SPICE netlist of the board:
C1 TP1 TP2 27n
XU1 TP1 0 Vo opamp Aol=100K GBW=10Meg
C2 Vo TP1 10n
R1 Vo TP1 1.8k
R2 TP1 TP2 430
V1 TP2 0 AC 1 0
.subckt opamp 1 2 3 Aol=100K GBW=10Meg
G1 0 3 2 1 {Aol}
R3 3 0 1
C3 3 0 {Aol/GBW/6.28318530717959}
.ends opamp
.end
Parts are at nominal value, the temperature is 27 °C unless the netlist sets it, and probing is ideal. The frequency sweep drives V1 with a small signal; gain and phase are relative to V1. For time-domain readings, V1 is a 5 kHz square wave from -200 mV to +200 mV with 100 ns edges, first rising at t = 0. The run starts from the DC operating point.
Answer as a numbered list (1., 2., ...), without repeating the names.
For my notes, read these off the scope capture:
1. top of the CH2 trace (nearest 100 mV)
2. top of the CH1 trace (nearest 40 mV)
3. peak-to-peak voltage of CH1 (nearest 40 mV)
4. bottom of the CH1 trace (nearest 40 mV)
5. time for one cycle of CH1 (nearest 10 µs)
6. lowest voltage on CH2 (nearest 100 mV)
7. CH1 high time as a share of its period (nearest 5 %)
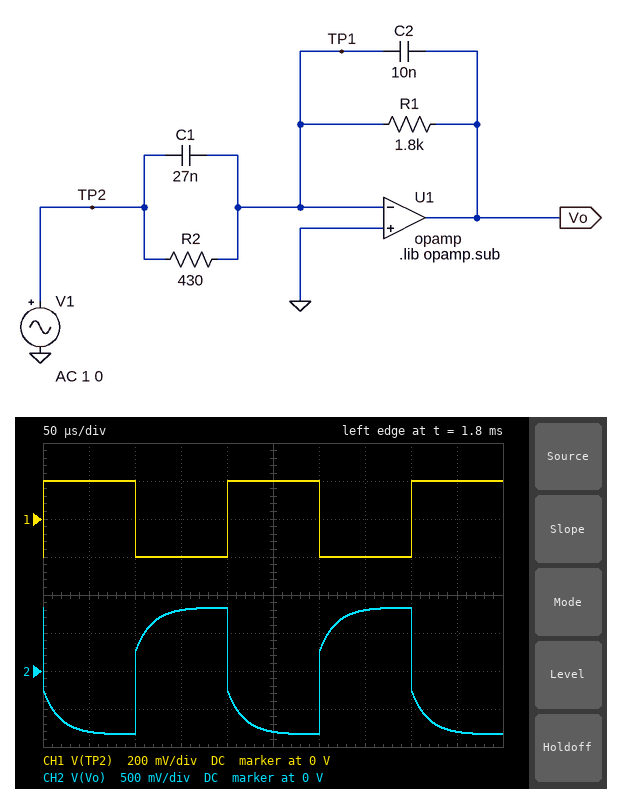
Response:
1. 800 mV
2. 200 mV
3. 400 mV
4. -200 mV
5. 200 µs
6. -800 mV
7. 50 %
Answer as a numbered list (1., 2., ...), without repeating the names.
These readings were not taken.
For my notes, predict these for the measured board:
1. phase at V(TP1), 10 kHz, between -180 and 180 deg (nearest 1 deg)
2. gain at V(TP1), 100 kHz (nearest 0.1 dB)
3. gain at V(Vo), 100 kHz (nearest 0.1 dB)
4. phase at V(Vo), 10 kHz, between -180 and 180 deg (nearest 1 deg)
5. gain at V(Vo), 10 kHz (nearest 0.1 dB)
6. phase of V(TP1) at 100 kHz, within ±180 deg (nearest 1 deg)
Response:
1. 77 deg
2. -31.3 dB
3. 8.7 dB
4. 167 deg
5. 10.7 dB
6. 85 deg
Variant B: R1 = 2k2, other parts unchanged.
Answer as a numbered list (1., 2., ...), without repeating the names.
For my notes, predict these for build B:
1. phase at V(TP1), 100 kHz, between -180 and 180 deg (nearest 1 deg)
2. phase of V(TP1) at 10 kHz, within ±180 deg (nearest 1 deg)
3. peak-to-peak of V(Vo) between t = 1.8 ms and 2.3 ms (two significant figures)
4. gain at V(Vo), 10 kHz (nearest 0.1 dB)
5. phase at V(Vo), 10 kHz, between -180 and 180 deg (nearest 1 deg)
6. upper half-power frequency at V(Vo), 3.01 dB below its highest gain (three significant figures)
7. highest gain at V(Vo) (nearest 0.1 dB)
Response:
1. 84 deg
2. 71 deg
3. 2.0 V
4. 11.4 dB
5. 162 deg
6. 10.8 kHz
7. 14.2 dB
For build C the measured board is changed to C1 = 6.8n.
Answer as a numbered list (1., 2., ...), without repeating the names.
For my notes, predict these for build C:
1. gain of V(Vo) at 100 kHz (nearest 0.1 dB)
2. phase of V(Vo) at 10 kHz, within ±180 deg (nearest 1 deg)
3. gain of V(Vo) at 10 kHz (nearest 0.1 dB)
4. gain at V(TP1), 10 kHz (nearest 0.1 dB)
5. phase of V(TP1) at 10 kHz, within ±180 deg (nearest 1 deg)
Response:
1. -2.3 dB
2. 142 deg
3. 9.0 dB
4. -51.0 dB
5. 51 deg
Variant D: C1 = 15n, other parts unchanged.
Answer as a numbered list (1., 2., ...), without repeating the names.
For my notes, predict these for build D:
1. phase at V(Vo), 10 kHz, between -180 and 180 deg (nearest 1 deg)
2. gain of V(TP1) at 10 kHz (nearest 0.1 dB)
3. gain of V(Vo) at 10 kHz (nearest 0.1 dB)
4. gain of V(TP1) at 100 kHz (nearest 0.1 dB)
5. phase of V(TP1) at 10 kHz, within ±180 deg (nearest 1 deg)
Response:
1. 153 deg
2. -50.5 dB
3. 9.5 dB
4. -36.3 dB
5. 63 deg
